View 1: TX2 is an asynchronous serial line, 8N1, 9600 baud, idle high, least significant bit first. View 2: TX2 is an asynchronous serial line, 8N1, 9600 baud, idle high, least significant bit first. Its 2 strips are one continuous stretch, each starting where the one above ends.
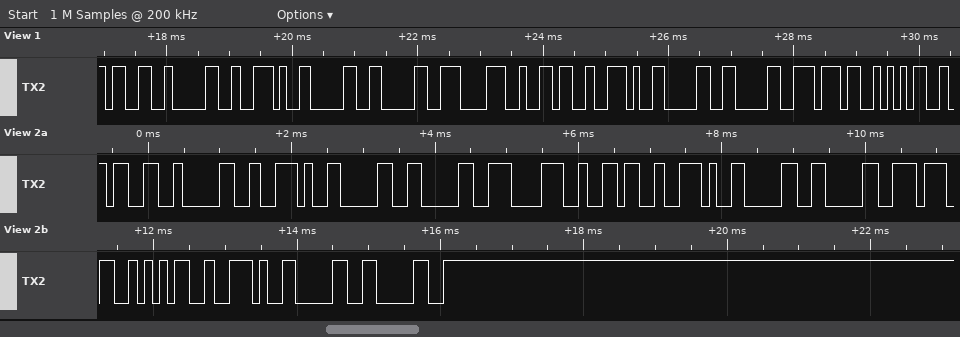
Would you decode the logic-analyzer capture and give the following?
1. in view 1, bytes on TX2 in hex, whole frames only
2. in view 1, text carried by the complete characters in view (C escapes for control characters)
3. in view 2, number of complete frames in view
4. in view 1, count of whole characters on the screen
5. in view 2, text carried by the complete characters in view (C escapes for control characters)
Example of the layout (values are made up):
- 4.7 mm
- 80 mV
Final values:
- 33 30 2E 30 30 38 36 2E 30 30 37 35
- "30.0086.0075"
- 15
- 12
- "30.0086.0075.00"
